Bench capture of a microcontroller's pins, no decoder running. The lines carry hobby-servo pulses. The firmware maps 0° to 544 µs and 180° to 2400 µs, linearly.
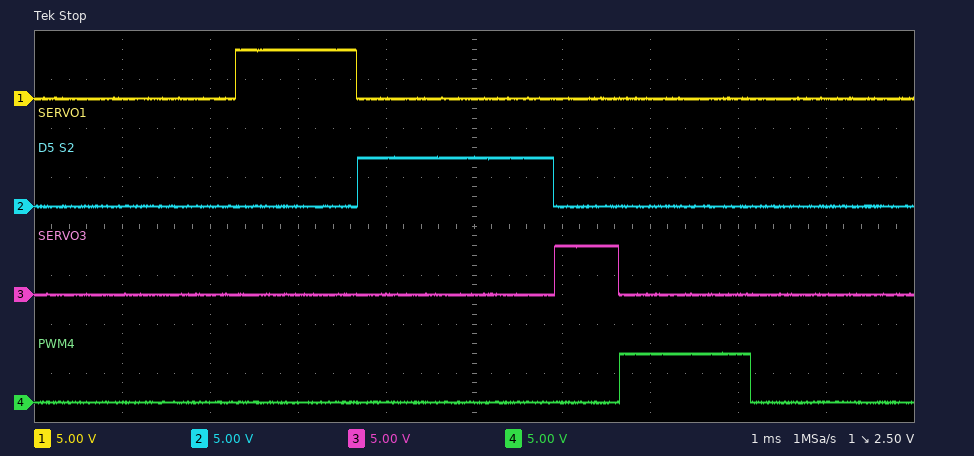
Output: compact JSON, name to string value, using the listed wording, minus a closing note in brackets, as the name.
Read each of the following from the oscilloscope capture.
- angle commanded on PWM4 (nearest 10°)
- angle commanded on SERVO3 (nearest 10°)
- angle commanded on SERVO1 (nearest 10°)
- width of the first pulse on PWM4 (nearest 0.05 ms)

{"angle commanded on PWM4": "90°", "angle commanded on SERVO3": "20°", "angle commanded on SERVO1": "80°", "width of the first pulse on PWM4": "1.50 ms"}
